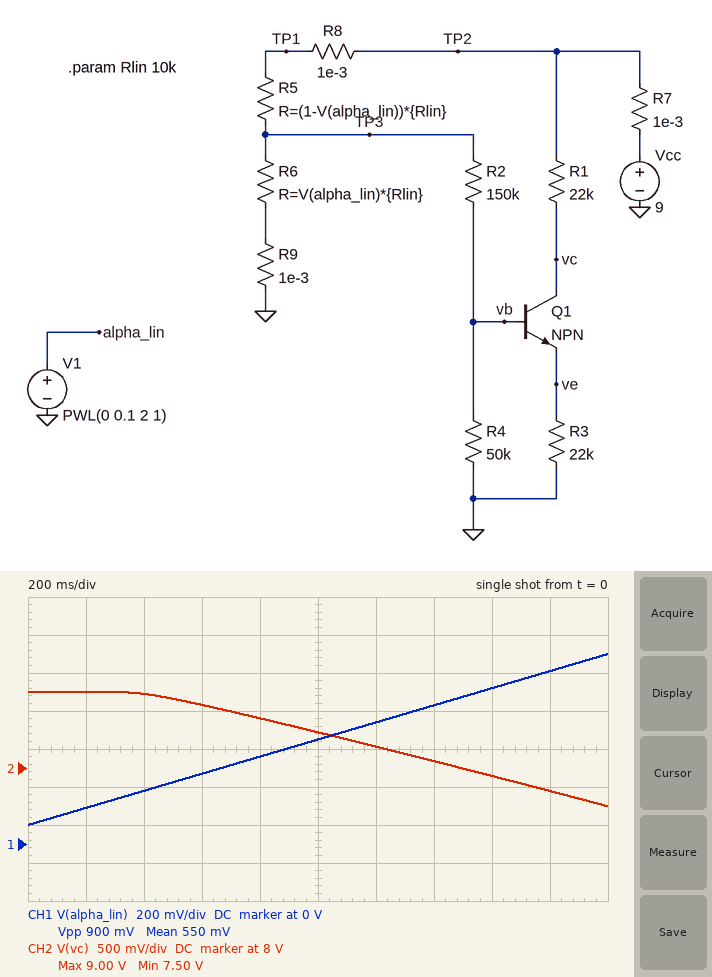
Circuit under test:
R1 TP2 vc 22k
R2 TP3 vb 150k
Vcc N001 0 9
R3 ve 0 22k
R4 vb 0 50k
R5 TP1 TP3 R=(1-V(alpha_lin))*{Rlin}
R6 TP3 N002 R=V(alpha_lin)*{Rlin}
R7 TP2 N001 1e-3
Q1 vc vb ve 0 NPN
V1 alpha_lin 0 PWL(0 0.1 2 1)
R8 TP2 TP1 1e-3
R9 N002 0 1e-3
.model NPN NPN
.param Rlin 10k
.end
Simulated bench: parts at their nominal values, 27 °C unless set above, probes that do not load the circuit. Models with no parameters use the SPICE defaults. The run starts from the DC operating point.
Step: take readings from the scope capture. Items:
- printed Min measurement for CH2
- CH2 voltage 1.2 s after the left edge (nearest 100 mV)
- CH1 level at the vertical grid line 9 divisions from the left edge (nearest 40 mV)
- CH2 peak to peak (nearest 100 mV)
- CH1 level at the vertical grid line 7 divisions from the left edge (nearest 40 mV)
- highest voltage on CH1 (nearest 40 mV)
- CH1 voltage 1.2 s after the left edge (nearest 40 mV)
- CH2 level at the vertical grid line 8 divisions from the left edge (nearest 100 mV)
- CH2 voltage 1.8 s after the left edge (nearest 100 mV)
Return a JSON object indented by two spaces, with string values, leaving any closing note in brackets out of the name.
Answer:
{
  "printed Min measurement for CH2": "7.50 V",
  "CH2 voltage 1.2 s after the left edge": "8.3 V",
  "CH1 level at the vertical grid line 9 divisions from the left edge": "920 mV",
  "CH2 peak to peak": "1.5 V",
  "CH1 level at the vertical grid line 7 divisions from the left edge": "720 mV",
  "highest voltage on CH1": "1.00 V",
  "CH1 voltage 1.2 s after the left edge": "640 mV",
  "CH2 level at the vertical grid line 8 divisions from the left edge": "7.9 V",
  "CH2 voltage 1.8 s after the left edge": "7.7 V"
}
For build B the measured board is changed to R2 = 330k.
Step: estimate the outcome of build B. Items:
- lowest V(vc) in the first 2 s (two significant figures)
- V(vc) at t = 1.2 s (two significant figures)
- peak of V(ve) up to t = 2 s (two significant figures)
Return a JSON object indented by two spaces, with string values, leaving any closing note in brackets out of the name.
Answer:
{
  "lowest V(vc) in the first 2 s": "8.5 V",
  "V(vc) at t = 1.2 s": "8.9 V",
  "peak of V(ve) up to t = 2 s": "500 mV"
}
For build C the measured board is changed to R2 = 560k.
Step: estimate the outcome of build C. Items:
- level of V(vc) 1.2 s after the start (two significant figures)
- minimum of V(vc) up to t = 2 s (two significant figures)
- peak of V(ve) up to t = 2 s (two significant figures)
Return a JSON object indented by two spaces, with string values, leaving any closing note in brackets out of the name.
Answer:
{
  "level of V(vc) 1.2 s after the start": "9.0 V",
  "minimum of V(vc) up to t = 2 s": "8.9 V",
  "peak of V(ve) up to t = 2 s": "100 mV"
}
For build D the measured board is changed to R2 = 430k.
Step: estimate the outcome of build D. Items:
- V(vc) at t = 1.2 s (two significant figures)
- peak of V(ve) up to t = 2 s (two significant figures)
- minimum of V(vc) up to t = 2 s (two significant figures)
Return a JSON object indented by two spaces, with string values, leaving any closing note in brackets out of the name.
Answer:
{
  "V(vc) at t = 1.2 s": "9.0 V",
  "peak of V(ve) up to t = 2 s": "270 mV",
  "minimum of V(vc) up to t = 2 s": "8.7 V"
}
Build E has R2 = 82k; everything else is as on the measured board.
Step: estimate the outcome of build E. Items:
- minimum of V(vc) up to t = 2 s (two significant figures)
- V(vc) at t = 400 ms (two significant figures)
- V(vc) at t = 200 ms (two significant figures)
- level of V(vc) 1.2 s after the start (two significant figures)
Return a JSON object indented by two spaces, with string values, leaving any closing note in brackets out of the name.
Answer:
{
  "minimum of V(vc) up to t = 2 s": "6.4 V",
  "V(vc) at t = 400 ms": "8.7 V",
  "V(vc) at t = 200 ms": "9.0 V",
  "level of V(vc) 1.2 s after the start": "7.6 V"
}
